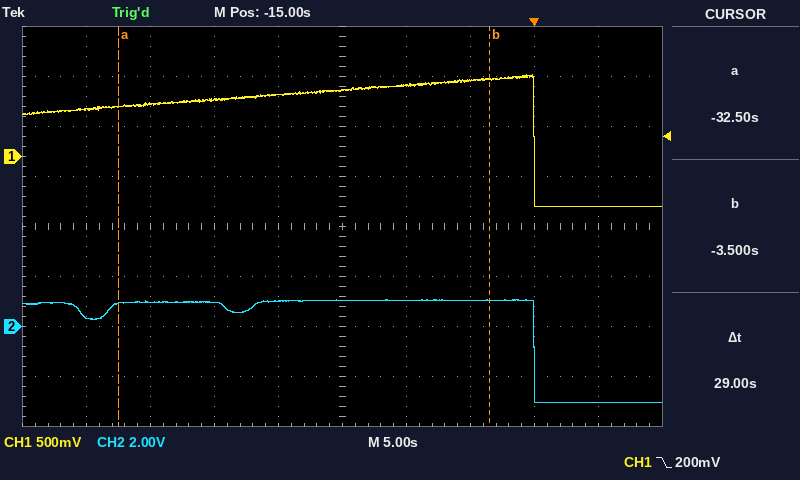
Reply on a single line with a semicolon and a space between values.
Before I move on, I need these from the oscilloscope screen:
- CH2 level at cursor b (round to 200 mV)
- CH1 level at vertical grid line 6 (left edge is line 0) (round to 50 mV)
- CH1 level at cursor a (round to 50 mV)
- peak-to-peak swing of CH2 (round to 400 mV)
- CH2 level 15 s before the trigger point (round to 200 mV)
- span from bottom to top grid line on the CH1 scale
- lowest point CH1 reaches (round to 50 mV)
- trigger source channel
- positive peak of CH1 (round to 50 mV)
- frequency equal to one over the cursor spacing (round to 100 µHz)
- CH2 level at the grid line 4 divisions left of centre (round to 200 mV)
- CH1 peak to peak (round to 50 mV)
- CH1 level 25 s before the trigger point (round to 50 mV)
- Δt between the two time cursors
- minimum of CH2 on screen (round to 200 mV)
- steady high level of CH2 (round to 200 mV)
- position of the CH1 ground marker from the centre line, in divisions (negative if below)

1.0 V; 700 mV; 500 mV; 4.0 V; 1.0 V; 4 V; -500 mV; CH1; 800 mV; 34.5 mHz; 400 mV; 1.30 V; 550 mV; 29 s; -3.0 V; 1.0 V; +1.4 div
